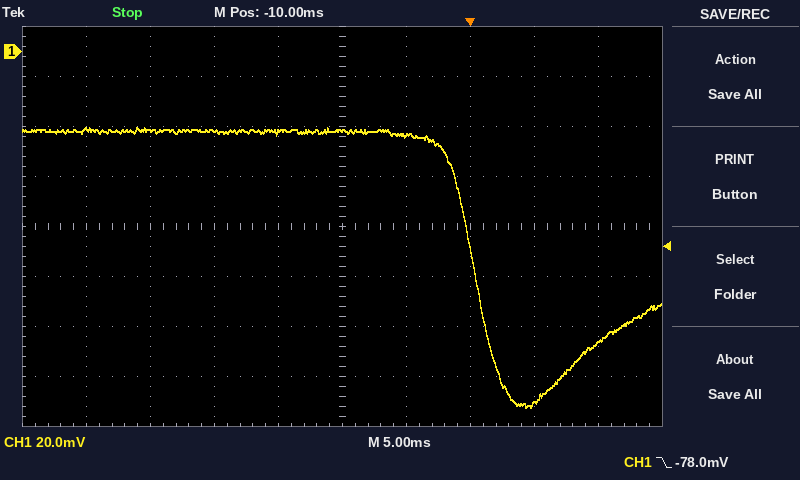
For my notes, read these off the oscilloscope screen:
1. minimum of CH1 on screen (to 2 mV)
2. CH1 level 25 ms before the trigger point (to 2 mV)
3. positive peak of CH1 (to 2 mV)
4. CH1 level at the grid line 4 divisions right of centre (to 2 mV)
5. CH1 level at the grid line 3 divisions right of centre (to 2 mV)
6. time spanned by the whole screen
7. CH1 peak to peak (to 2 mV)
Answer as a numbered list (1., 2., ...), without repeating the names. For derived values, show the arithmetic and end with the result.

1. -142 mV
2. -32 mV
3. -30 mV
4. -116 mV
5. -142 mV
6. 50 ms
7. -30 mV − (-142 mV) = 112 mV
